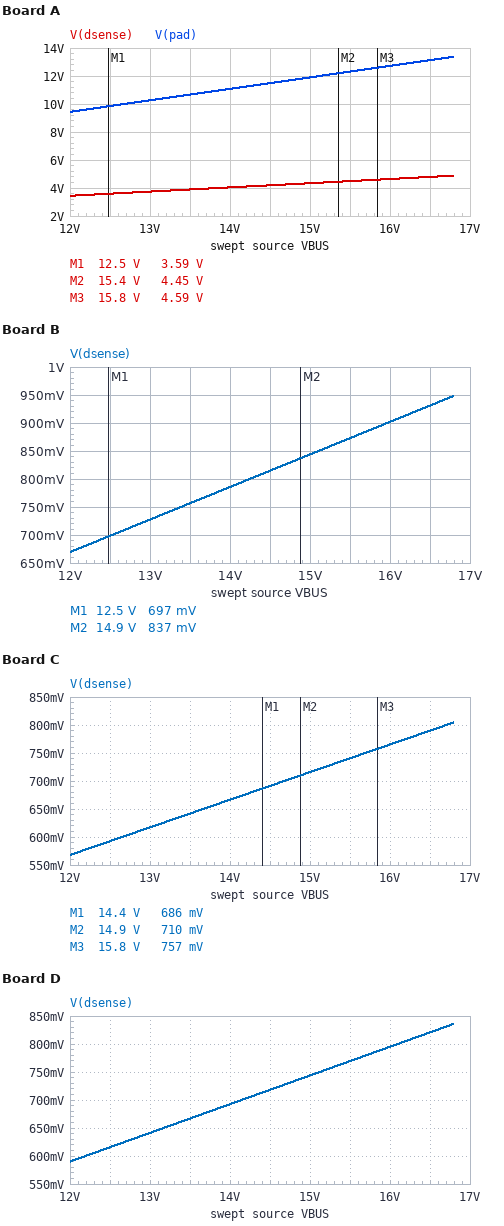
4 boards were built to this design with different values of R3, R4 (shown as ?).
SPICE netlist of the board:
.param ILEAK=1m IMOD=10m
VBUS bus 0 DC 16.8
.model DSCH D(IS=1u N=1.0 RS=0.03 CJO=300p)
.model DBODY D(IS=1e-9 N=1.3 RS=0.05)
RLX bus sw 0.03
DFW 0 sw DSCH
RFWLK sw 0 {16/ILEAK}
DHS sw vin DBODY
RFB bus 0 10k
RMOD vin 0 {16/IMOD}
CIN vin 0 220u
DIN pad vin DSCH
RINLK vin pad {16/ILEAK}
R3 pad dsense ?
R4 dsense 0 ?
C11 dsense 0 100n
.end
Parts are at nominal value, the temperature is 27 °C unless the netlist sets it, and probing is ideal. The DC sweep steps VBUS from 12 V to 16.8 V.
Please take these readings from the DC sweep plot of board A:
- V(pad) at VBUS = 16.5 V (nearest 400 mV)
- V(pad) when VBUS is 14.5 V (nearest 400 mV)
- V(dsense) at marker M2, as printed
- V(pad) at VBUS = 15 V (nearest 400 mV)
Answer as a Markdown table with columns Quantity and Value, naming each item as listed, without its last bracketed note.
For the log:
| Quantity | Value |
|---|---|
| V(pad) at VBUS = 16.5 V | 13.2 V |
| V(pad) when VBUS is 14.5 V | 11.6 V |
| V(dsense) at marker M2, as printed | 4.45 V |
| V(pad) at VBUS = 15 V | 12.0 V |
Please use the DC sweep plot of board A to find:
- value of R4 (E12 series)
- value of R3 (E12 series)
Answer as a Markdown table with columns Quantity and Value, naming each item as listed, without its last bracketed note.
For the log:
| Quantity | Value |
|---|---|
| value of R4 | 27 kΩ |
| value of R3 | 47 kΩ |
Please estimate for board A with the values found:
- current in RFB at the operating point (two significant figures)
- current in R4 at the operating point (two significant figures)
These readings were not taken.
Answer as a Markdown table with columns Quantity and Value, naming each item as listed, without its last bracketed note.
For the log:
| Quantity | Value |
|---|---|
| current in RFB at the operating point | 1.7 mA |
| current in R4 at the operating point | 180 µA |
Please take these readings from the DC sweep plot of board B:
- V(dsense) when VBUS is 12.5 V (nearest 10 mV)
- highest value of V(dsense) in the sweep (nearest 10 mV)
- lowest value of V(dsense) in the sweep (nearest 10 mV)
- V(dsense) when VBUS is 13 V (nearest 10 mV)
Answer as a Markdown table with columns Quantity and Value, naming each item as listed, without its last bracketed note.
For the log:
| Quantity | Value |
|---|---|
| V(dsense) when VBUS is 12.5 V | 700 mV |
| highest value of V(dsense) in the sweep | 950 mV |
| lowest value of V(dsense) in the sweep | 670 mV |
| V(dsense) when VBUS is 13 V | 730 mV |
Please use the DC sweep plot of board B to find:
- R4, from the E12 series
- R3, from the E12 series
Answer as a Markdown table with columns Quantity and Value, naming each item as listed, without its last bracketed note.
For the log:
| Quantity | Value |
|---|---|
| R4, from the E12 series | 3.9 kΩ |
| R3, from the E12 series | 47 kΩ |
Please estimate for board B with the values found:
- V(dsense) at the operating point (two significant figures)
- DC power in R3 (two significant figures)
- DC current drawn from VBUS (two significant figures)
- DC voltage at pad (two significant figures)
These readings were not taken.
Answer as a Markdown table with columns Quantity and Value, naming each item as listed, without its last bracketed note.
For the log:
| Quantity | Value |
|---|---|
| V(dsense) at the operating point | 950 mV |
| DC power in R3 | 2.8 mW |
| DC current drawn from VBUS | 13 mA |
| DC voltage at pad | 12 V |
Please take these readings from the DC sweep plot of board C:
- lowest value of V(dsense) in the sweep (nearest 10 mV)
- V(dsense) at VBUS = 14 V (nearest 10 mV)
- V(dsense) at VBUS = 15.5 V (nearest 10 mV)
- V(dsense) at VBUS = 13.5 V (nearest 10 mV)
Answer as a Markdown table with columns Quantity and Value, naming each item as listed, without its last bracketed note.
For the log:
| Quantity | Value |
|---|---|
| lowest value of V(dsense) in the sweep | 570 mV |
| V(dsense) at VBUS = 14 V | 670 mV |
| V(dsense) at VBUS = 15.5 V | 740 mV |
| V(dsense) at VBUS = 13.5 V | 640 mV |
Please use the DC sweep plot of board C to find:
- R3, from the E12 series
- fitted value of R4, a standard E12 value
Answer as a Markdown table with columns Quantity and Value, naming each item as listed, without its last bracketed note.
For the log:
| Quantity | Value |
|---|---|
| R3, from the E12 series | 330 kΩ |
| fitted value of R4, a standard E12 value | 18 kΩ |
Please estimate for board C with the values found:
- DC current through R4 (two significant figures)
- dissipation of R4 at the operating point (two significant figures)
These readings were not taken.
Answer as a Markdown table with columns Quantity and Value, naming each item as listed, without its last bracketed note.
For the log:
| Quantity | Value |
|---|---|
| DC current through R4 | 45 µA |
| dissipation of R4 at the operating point | 36 µW |
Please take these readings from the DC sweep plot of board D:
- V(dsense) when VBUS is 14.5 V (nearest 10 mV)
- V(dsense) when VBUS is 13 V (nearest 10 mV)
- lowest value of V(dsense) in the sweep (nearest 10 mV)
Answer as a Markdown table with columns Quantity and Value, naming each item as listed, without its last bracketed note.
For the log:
| Quantity | Value |
|---|---|
| V(dsense) when VBUS is 14.5 V | 720 mV |
| V(dsense) when VBUS is 13 V | 640 mV |
| lowest value of V(dsense) in the sweep | 590 mV |
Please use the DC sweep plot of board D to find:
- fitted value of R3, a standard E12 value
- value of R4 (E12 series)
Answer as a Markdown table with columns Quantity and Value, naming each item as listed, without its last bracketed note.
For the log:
| Quantity | Value |
|---|---|
| fitted value of R3, a standard E12 value | 56 kΩ |
| value of R4 | 3.9 kΩ |
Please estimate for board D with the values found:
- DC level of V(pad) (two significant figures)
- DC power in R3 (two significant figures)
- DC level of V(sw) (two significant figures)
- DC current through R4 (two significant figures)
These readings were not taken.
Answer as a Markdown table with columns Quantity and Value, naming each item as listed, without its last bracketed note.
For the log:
| Quantity | Value |
|---|---|
| DC level of V(pad) | 13 V |
| DC power in R3 | 2.6 mW |
| DC level of V(sw) | 17 V |
| DC current through R4 | 210 µA |
